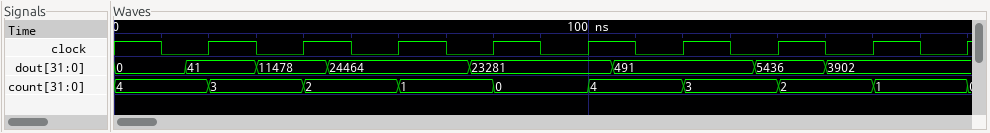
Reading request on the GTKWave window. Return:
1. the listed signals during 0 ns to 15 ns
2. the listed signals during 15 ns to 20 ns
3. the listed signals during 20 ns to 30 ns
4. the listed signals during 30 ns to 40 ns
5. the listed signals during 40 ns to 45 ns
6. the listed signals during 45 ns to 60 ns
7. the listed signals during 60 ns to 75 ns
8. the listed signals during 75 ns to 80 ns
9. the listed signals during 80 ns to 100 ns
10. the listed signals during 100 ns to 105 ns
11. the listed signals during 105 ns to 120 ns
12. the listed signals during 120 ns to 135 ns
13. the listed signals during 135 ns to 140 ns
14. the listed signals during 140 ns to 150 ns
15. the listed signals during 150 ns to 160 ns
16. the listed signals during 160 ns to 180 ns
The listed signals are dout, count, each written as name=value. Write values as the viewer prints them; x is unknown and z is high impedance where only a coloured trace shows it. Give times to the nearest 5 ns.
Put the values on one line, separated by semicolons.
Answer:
dout=0, count=4; dout=41, count=4; dout=41, count=3; dout=11478, count=3; dout=11478, count=2; dout=24464, count=2; dout=24464, count=1; dout=23281, count=1; dout=23281, count=0; dout=23281, count=4; dout=491, count=4; dout=491, count=3; dout=5436, count=3; dout=5436, count=2; dout=3902, count=2; dout=3902, count=1
